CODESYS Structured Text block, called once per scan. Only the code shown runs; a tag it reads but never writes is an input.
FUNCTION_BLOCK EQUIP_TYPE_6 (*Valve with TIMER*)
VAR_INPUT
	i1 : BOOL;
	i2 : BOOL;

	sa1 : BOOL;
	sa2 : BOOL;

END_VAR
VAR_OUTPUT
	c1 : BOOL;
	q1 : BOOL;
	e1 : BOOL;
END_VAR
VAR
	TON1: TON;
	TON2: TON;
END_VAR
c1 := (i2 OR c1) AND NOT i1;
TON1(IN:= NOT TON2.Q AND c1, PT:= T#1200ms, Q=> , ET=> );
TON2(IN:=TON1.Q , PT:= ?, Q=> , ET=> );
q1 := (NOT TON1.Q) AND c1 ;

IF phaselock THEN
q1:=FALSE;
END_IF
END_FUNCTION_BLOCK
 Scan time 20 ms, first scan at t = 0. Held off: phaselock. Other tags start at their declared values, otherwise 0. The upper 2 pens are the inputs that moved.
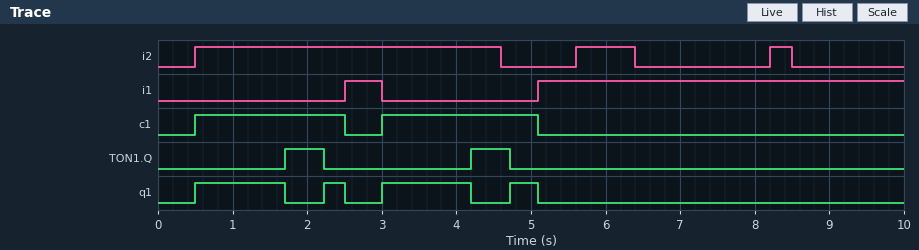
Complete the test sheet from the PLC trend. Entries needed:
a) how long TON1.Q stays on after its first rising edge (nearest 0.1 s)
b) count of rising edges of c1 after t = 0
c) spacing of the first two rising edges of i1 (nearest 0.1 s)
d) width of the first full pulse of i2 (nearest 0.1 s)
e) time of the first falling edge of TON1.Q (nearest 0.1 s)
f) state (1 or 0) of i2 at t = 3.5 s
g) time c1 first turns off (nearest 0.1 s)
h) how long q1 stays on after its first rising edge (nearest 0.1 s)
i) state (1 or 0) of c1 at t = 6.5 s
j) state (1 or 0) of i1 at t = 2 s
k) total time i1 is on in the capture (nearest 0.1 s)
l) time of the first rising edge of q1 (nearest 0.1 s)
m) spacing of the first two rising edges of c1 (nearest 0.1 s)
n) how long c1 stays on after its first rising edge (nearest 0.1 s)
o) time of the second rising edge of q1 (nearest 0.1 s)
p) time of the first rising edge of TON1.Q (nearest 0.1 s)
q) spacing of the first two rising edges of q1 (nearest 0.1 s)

0.5 s
2
2.6 s
4.1 s
2.2 s
1
2.5 s
1.2 s
0
0
5.4 s
0.5 s
2.5 s
2.0 s
2.2 s
1.7 s
1.7 s
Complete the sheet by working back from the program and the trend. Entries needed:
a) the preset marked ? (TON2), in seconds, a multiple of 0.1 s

0.5 s
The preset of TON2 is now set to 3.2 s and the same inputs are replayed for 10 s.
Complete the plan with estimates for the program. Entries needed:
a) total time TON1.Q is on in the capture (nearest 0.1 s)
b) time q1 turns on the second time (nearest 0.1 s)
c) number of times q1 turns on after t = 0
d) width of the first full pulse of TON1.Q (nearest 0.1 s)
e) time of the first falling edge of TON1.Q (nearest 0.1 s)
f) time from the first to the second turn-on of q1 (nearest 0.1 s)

1.7 s
3.0 s
2
0.8 s
2.5 s
2.5 s
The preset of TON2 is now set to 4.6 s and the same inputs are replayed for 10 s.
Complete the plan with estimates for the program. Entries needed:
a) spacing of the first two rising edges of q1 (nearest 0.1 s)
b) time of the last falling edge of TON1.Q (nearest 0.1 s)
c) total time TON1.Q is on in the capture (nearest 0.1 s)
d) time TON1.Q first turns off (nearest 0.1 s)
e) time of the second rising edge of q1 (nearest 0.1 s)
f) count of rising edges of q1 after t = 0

2.5 s
5.1 s
1.7 s
2.5 s
3.0 s
2
